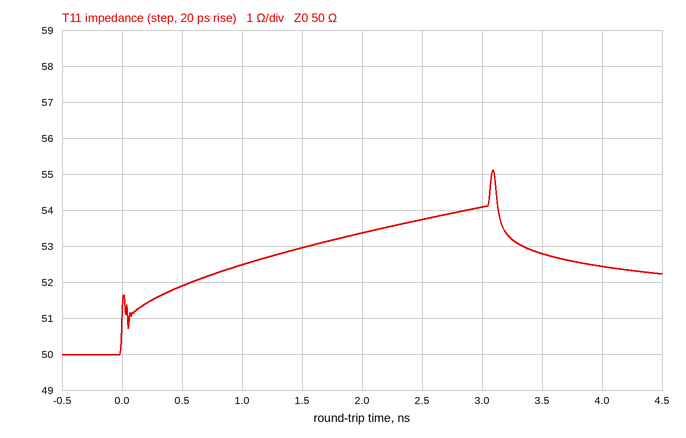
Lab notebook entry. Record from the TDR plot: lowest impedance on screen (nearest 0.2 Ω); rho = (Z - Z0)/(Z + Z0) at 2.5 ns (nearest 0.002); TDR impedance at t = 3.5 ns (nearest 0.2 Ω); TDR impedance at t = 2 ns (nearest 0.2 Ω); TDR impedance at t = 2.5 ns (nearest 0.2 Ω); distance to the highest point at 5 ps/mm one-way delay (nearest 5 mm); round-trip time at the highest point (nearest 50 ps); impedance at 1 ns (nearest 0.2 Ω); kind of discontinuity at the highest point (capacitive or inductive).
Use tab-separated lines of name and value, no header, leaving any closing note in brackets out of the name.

lowest impedance on screen	50.0 Ω
rho = (Z - Z0)/(Z + Z0) at 2.5 ns	+0.036
TDR impedance at t = 3.5 ns	52.8 Ω
TDR impedance at t = 2 ns	53.4 Ω
TDR impedance at t = 2.5 ns	53.8 Ω
distance to the highest point at 5 ps/mm one-way delay	310 mm
round-trip time at the highest point	3.10 ns
impedance at 1 ns	52.4 Ω
kind of discontinuity at the highest point	inductive
